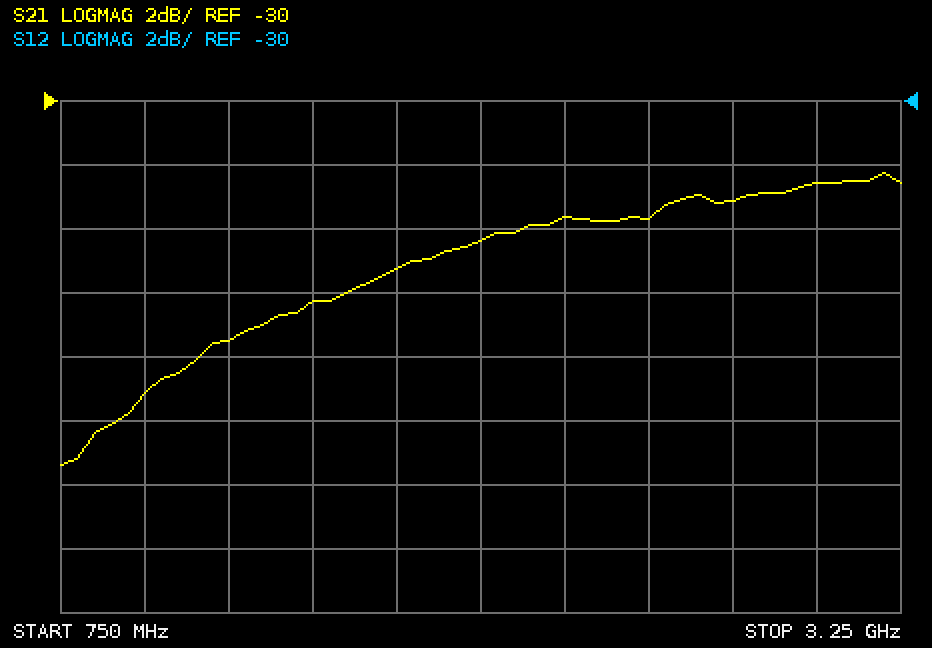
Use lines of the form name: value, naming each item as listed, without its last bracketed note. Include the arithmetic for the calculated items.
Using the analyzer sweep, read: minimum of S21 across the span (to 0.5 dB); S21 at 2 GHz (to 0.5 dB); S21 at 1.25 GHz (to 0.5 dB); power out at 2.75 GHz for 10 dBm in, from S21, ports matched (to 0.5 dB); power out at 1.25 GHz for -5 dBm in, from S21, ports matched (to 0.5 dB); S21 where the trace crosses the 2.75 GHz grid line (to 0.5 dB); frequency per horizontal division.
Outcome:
minimum of S21 across the span: -41.5 dB
S21 at 2 GHz: -34.5 dB
S21 at 1.25 GHz: -37.5 dB
power out at 2.75 GHz for 10 dBm in, from S21, ports matched: 10 dBm + (-33.0 dB) = -23.0 dBm
power out at 1.25 GHz for -5 dBm in, from S21, ports matched: -5 dBm + (-37.5 dB) = -42.5 dBm
S21 where the trace crosses the 2.75 GHz grid line: -33.0 dB
frequency per horizontal division: 250 MHz
